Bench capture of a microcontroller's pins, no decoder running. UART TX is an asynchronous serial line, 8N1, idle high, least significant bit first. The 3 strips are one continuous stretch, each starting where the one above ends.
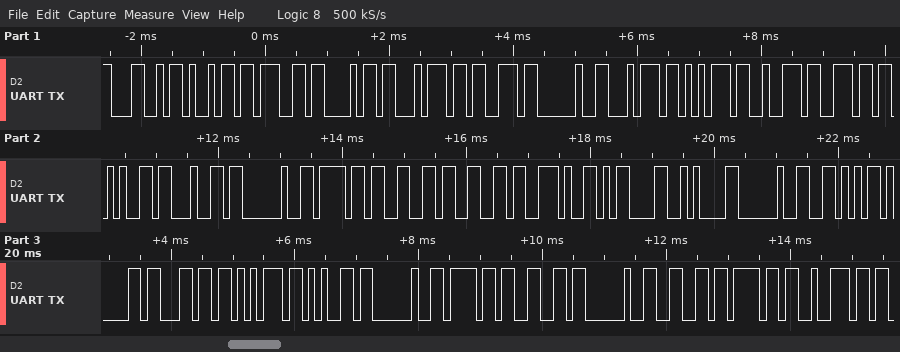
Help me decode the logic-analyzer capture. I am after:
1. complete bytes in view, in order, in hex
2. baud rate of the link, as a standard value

4C 69 67 68 74 73 20 74 75 72 6E 65 64 20 6F 66 66 2E 0D 0A 20 56 61 6C 75 65 20 6F 66 20 66 6F 72
9600 baud
